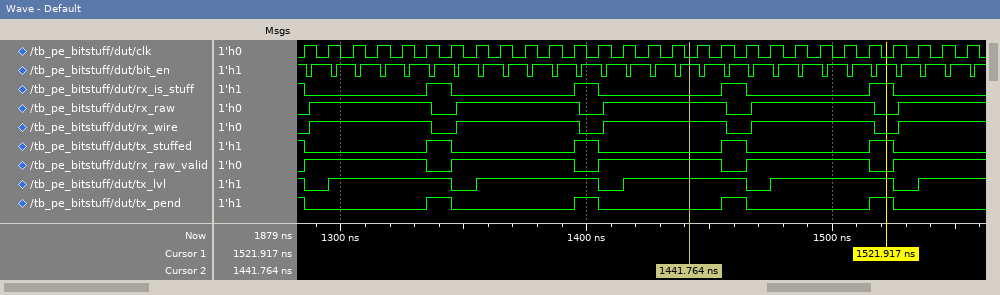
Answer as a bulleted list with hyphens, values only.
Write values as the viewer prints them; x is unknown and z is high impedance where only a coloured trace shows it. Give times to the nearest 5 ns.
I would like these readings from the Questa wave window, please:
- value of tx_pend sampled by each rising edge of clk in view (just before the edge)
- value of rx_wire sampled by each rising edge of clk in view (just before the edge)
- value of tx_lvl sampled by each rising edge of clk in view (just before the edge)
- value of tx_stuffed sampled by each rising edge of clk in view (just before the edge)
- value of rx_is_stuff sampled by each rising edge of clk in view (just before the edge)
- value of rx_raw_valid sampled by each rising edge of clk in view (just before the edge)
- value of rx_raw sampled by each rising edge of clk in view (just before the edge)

- 1 0 0 0 0 0 1 0 0 0 0 0 1 0 0 0 0 0 1 0 0 0 0 0 1 0 0 0
- 0 1 1 1 1 1 0 1 1 1 1 1 0 1 1 1 1 1 0 1 1 1 1 1 0 1 1 1
- 1 0 1 1 1 1 1 0 1 1 1 1 1 0 1 1 1 1 1 0 1 1 1 1 1 0 1 1
- 1 0 0 0 0 0 1 0 0 0 0 0 1 0 0 0 0 0 1 0 0 0 0 0 1 0 0 0
- 1 0 0 0 0 0 1 0 0 0 0 0 1 0 0 0 0 0 1 0 0 0 0 0 1 0 0 0
- 0 1 1 1 1 1 0 1 1 1 1 1 0 1 1 1 1 1 0 1 1 1 1 1 0 1 1 1
- 0 1 1 1 1 1 0 1 1 1 1 1 0 1 1 1 1 1 0 1 1 1 1 1 0 1 1 1
